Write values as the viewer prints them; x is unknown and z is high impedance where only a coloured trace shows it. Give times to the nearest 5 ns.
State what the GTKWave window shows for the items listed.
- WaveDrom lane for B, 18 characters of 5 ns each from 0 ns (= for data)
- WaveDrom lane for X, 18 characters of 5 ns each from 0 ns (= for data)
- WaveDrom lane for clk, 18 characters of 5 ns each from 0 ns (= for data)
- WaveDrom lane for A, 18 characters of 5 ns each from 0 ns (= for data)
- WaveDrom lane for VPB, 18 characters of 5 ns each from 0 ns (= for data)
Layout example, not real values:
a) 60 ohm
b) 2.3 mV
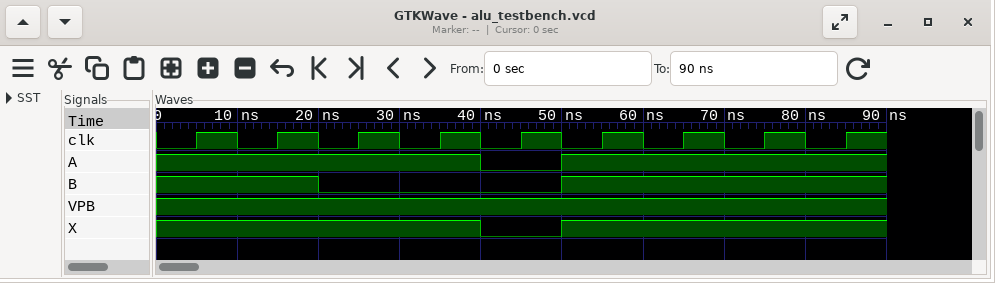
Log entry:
a) {name: 'B', wave: '1...0.....1.......'}
b) {name: 'X', wave: '1.......0.1.......'}
c) {name: 'clk', wave: '010101010101010101'}
d) {name: 'A', wave: '1.......0.1.......'}
e) {name: 'VPB', wave: '1.................'}
